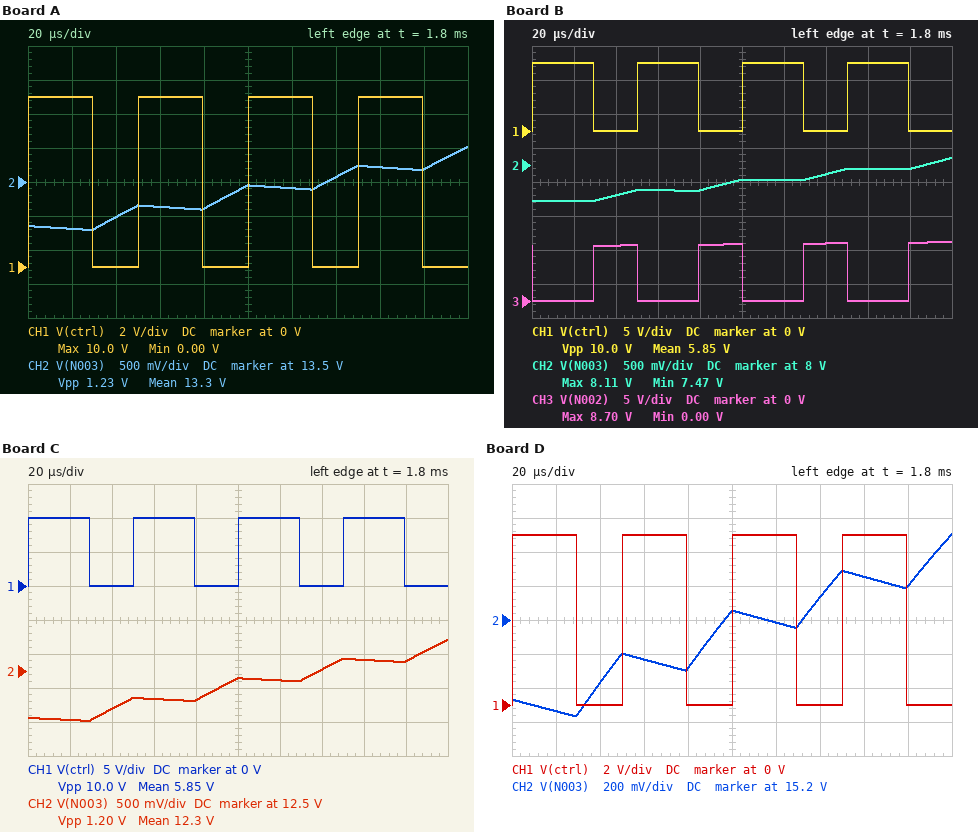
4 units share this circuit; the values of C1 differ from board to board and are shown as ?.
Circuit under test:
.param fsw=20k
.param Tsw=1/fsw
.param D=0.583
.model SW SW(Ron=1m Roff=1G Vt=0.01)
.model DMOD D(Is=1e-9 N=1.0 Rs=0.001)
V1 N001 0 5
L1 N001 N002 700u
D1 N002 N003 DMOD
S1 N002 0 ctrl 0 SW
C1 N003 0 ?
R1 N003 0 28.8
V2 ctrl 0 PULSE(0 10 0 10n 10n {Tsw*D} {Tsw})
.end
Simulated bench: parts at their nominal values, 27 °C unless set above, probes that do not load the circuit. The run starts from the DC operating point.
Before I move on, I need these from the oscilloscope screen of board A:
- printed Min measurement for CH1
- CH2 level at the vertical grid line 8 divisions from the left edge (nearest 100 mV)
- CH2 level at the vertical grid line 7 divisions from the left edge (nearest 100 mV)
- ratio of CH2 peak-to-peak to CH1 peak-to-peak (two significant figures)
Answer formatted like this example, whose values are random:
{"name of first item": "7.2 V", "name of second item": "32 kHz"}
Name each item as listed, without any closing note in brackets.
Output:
{"printed Min measurement for CH1": "0.00 V", "CH2 level at the vertical grid line 8 divisions from the left edge": "13.7 V", "CH2 level at the vertical grid line 7 divisions from the left edge": "13.6 V", "ratio of CH2 peak-to-peak to CH1 peak-to-peak": "0.12"}
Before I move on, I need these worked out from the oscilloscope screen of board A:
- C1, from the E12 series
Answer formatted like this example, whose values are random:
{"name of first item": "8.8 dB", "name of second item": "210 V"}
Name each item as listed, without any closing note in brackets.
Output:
{"C1, from the E12 series": "220 µF"}
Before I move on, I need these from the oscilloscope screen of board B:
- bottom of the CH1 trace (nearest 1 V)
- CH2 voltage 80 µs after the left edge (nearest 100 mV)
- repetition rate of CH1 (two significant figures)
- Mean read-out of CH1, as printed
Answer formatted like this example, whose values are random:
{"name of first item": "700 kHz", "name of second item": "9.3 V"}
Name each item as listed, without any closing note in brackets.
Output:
{"bottom of the CH1 trace": "0 V", "CH2 voltage 80 µs after the left edge": "7.6 V", "repetition rate of CH1": "20 kHz", "Mean read-out of CH1, as printed": "5.85 V"}
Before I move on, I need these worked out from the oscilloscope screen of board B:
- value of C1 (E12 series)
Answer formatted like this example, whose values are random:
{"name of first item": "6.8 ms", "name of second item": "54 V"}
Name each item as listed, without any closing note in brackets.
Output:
{"value of C1": "820 µF"}
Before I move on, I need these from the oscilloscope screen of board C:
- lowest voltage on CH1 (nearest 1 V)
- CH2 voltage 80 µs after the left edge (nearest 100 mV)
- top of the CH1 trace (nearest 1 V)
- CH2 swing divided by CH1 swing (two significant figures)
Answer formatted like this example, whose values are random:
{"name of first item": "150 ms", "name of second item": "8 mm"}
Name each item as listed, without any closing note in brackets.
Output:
{"lowest voltage on CH1": "0 V", "CH2 voltage 80 µs after the left edge": "12.1 V", "top of the CH1 trace": "10 V", "CH2 swing divided by CH1 swing": "0.12"}
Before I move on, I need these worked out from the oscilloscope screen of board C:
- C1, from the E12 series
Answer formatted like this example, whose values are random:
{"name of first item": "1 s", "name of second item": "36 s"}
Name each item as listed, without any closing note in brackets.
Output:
{"C1, from the E12 series": "270 µF"}
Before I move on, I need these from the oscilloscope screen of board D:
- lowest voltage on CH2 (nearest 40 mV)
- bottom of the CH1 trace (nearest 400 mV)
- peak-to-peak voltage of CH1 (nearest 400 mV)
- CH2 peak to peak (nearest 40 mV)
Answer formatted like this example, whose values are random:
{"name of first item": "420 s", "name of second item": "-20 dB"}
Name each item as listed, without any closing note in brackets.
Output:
{"lowest voltage on CH2": "14.64 V", "bottom of the CH1 trace": "0 V", "peak-to-peak voltage of CH1": "10.0 V", "CH2 peak to peak": "1.08 V"}
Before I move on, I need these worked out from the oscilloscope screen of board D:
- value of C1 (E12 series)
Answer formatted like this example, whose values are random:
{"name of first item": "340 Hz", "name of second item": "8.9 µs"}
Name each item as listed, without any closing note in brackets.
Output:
{"value of C1": "150 µF"}
